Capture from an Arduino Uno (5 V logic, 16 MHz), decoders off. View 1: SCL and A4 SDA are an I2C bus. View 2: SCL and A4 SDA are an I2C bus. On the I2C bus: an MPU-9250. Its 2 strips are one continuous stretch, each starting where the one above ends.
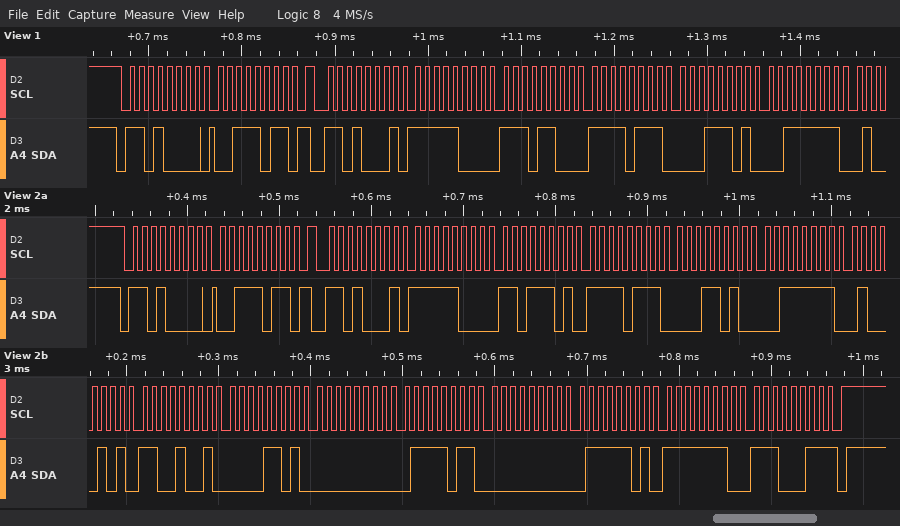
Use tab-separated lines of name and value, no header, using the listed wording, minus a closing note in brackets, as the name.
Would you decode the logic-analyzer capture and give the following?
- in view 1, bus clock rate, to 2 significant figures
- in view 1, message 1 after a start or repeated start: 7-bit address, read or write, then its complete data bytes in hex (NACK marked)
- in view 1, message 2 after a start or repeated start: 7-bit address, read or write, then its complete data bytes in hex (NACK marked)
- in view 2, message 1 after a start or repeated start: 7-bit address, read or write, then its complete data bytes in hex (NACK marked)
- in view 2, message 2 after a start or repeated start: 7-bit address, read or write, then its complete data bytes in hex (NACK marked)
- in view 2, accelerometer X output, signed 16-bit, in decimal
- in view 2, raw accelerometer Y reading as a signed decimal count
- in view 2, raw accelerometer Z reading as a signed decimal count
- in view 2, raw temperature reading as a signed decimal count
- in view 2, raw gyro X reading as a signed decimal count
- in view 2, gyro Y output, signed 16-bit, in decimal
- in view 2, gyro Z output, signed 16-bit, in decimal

in view 1, bus clock rate, to 2 significant figures	100 kHz
in view 1, message 1 after a start or repeated start: 7-bit address, read or write, then its complete data bytes in hex	0x68 write: 3B
in view 1, message 2 after a start or repeated start: 7-bit address, read or write, then its complete data bytes in hex	0x68 read: F8 EC F7 1D 3F
in view 2, message 1 after a start or repeated start: 7-bit address, read or write, then its complete data bytes in hex	0x68 write: 3B
in view 2, message 2 after a start or repeated start: 7-bit address, read or write, then its complete data bytes in hex	0x68 read: F8 DD F7 1A 3F 45 C9 0D 00 7B 00 7D FE E3 NACK
in view 2, accelerometer X output, signed 16-bit, in decimal	-1827
in view 2, raw accelerometer Y reading as a signed decimal count	-2278
in view 2, raw accelerometer Z reading as a signed decimal count	16197
in view 2, raw temperature reading as a signed decimal count	-14067
in view 2, raw gyro X reading as a signed decimal count	123
in view 2, gyro Y output, signed 16-bit, in decimal	125
in view 2, gyro Z output, signed 16-bit, in decimal	-285
